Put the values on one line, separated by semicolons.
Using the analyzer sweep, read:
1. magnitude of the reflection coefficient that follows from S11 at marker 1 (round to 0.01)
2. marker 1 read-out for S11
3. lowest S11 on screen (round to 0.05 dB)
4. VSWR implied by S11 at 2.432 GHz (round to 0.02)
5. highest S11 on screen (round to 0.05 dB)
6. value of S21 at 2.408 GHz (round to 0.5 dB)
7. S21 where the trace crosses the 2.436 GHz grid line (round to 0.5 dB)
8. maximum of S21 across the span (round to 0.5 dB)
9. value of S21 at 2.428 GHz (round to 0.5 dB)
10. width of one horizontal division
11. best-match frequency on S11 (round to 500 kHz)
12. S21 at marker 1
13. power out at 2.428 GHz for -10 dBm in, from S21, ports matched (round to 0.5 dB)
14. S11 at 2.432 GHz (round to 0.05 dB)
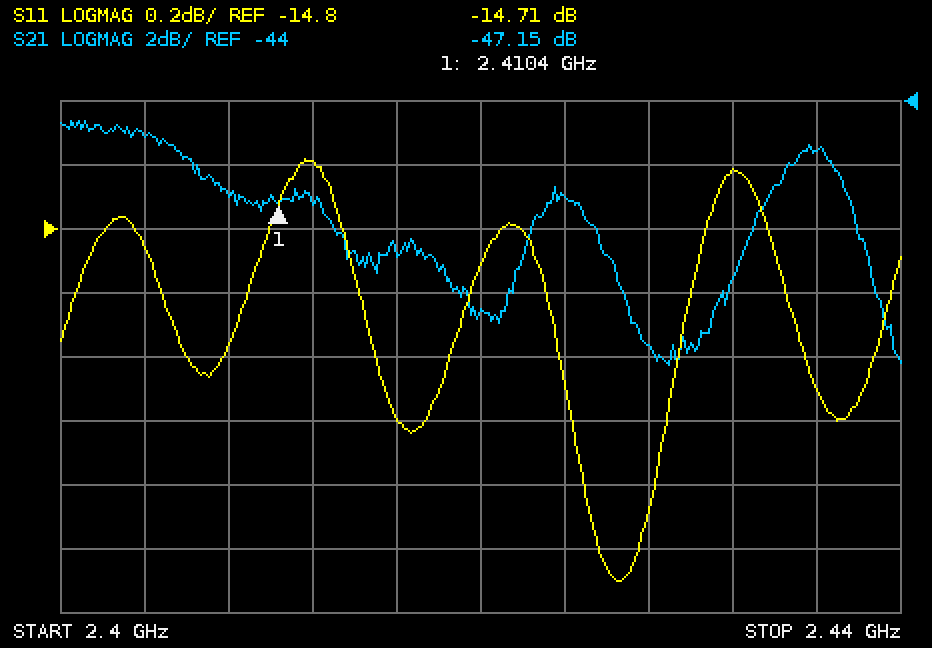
0.18; -14.71 dB; -15.90 dB; 1.46; -14.60 dB; -47.0 dB; -45.5 dB; -44.5 dB; -51.5 dB; 4 MHz; 2.4265 GHz; -47.15 dB; -61.5 dBm; -14.60 dB
